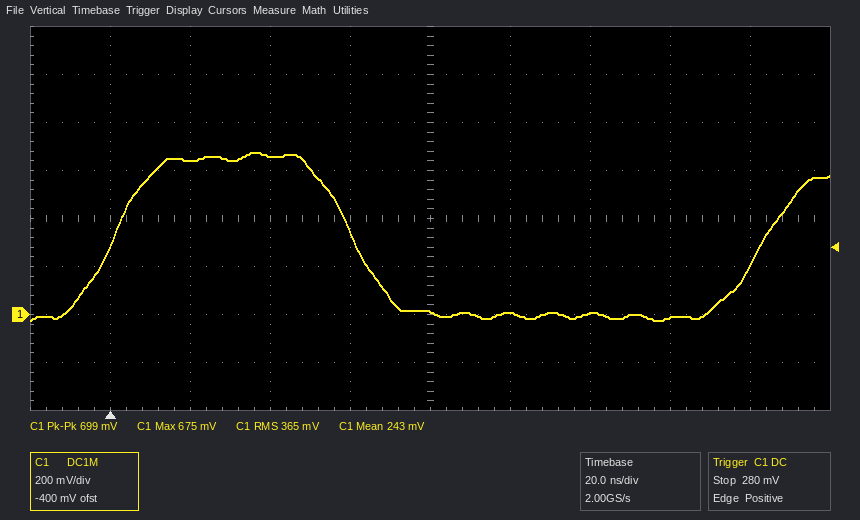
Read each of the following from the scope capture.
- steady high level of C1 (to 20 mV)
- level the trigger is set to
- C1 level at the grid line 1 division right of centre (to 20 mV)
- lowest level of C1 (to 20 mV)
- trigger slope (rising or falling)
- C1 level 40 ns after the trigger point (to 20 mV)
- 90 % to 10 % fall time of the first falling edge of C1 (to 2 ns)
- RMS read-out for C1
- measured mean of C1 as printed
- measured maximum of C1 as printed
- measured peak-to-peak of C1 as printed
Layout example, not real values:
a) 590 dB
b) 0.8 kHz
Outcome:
a) 660 mV
b) 280 mV
c) 0 mV
d) -20 mV
e) rising
f) 660 mV
g) 20 ns
h) 365 mV
i) 243 mV
j) 675 mV
k) 699 mV
